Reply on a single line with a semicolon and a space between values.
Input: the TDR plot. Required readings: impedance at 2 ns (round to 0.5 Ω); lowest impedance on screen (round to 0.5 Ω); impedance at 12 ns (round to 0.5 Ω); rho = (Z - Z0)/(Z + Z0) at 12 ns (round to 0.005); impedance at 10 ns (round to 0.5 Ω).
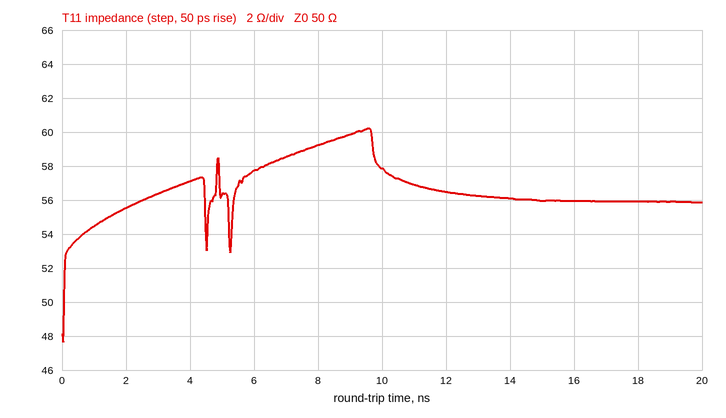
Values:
55.5 Ω; 47.5 Ω; 56.5 Ω; +0.060; 58.0 Ω
